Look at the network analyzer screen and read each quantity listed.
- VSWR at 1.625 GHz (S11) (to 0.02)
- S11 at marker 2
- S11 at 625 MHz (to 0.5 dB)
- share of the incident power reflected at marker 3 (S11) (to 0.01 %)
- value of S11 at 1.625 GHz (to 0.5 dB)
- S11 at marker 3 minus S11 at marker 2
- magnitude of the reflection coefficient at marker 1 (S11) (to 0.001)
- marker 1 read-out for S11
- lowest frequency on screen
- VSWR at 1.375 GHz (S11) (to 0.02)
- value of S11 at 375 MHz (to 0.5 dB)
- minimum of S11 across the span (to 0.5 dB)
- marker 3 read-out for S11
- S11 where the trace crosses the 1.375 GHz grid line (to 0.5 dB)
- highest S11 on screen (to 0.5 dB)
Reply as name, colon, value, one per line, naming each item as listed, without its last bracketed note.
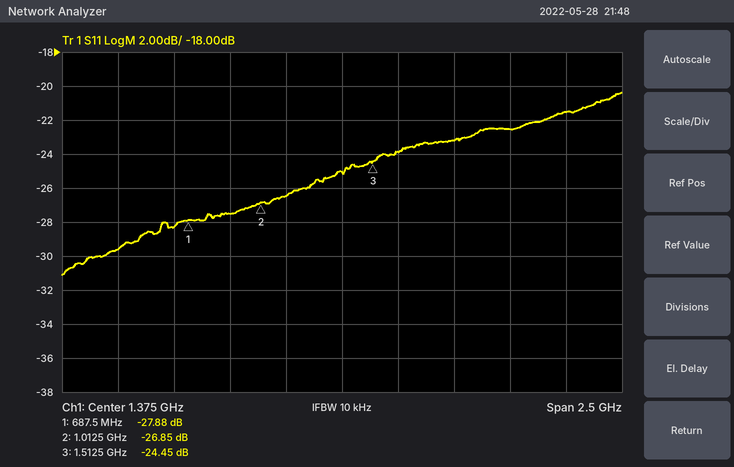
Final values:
VSWR at 1.625 GHz (S11): 1.14
S11 at marker 2: -26.85 dB
S11 at 625 MHz: -28.5 dB
share of the incident power reflected at marker 3 (S11): 0.36 %
value of S11 at 1.625 GHz: -24.0 dB
S11 at marker 3 minus S11 at marker 2: 2.40 dB
magnitude of the reflection coefficient at marker 1 (S11): 0.040
marker 1 read-out for S11: -27.88 dB
lowest frequency on screen: 125 MHz
VSWR at 1.375 GHz (S11): 1.12
value of S11 at 375 MHz: -29.5 dB
minimum of S11 across the span: -31.0 dB
marker 3 read-out for S11: -24.45 dB
S11 where the trace crosses the 1.375 GHz grid line: -25.0 dB
highest S11 on screen: -20.5 dB
